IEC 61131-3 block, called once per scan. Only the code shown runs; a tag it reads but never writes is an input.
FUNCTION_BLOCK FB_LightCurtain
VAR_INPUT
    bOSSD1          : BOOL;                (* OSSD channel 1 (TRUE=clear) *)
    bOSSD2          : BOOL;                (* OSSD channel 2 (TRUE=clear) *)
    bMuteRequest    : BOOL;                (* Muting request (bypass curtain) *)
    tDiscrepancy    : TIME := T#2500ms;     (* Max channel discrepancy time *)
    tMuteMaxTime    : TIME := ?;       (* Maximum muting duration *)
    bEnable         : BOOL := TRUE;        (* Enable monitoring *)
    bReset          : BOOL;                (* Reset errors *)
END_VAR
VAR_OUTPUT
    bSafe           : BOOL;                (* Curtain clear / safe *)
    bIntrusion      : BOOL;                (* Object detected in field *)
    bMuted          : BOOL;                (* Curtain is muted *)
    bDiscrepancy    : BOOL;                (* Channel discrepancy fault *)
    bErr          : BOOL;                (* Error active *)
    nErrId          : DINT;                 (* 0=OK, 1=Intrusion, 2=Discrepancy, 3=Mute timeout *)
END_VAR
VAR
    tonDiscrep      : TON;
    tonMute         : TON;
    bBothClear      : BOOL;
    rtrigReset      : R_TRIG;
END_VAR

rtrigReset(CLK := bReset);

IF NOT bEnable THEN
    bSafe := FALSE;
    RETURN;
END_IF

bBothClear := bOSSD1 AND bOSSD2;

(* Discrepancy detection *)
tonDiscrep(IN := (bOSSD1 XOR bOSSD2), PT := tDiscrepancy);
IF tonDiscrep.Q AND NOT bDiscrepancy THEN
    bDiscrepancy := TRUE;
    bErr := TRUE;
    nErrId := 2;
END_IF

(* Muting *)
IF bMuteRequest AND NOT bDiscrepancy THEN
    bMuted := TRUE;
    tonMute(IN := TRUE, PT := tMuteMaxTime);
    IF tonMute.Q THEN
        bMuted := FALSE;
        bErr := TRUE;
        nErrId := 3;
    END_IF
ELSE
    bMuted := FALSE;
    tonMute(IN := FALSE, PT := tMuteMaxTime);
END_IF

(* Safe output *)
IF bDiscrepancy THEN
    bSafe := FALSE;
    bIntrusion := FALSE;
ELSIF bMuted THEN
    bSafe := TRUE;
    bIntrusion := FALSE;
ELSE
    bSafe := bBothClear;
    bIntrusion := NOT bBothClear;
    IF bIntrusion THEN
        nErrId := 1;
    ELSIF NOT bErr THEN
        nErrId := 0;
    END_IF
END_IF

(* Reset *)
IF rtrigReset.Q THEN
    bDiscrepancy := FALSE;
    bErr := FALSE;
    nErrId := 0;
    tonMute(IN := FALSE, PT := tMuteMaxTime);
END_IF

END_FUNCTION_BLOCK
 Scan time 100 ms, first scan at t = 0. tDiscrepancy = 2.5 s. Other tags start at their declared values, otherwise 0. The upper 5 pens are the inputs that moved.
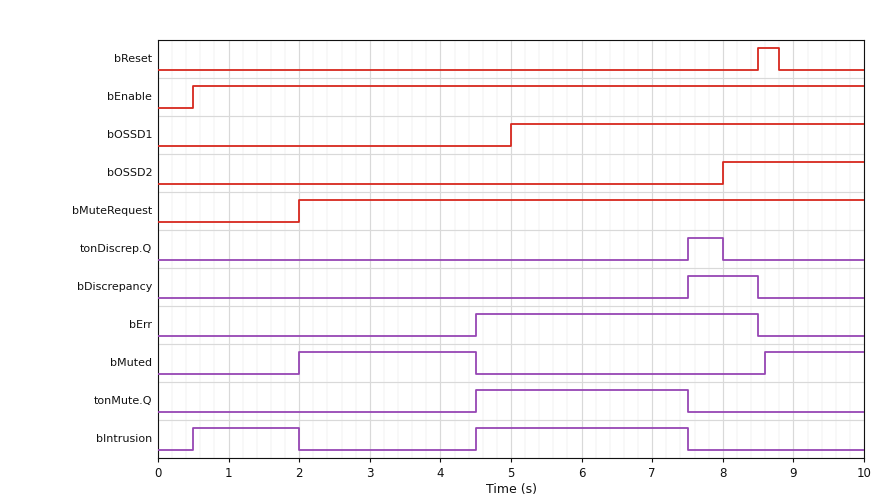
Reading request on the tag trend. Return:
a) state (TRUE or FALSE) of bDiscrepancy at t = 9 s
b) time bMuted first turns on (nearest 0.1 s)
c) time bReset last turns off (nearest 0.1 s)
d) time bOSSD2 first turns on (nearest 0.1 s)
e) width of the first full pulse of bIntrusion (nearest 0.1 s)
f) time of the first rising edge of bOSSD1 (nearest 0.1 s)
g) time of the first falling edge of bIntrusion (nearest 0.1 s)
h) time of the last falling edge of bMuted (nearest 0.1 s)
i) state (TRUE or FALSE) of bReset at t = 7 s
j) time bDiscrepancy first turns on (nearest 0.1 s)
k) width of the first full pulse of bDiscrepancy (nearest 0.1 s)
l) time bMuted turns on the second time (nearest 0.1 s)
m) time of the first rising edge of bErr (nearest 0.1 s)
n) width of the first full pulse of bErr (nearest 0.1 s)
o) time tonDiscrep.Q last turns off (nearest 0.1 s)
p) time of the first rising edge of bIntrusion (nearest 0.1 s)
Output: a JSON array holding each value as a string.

["FALSE", "2.0 s", "8.8 s", "8.0 s", "1.5 s", "5.0 s", "2.0 s", "4.5 s", "FALSE", "7.5 s", "1.0 s", "8.6 s", "4.5 s", "4.0 s", "8.0 s", "0.5 s"]
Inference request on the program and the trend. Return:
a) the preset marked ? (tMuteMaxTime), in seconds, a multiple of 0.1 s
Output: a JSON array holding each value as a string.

["2.5 s"]
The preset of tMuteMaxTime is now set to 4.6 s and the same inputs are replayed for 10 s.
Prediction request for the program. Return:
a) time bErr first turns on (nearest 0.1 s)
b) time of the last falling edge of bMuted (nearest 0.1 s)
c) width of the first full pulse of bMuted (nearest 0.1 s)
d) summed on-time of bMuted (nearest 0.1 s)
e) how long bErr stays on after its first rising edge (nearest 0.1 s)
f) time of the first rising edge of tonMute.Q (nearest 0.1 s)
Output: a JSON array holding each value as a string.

["6.6 s", "6.6 s", "4.6 s", "6.0 s", "1.9 s", "6.6 s"]
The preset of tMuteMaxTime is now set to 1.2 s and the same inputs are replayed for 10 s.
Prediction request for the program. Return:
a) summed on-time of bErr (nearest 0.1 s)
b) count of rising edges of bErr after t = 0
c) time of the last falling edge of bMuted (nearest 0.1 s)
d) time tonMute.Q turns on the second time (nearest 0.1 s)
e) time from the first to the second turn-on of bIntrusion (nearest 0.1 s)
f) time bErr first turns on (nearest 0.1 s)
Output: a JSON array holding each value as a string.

["5.5 s", "2", "9.8 s", "9.8 s", "2.7 s", "3.2 s"]
